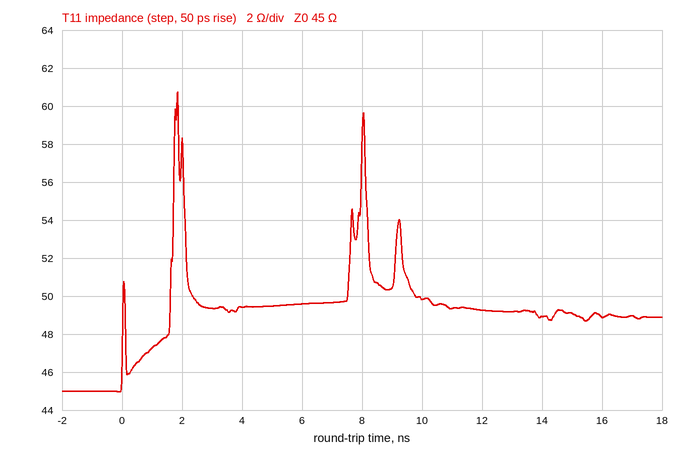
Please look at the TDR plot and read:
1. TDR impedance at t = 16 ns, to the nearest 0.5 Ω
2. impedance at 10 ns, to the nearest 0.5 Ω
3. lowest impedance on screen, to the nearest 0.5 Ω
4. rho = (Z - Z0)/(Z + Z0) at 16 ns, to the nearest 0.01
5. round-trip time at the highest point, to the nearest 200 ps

49.0 Ω
50.0 Ω
45.0 Ω
+0.04
1.8 ns
